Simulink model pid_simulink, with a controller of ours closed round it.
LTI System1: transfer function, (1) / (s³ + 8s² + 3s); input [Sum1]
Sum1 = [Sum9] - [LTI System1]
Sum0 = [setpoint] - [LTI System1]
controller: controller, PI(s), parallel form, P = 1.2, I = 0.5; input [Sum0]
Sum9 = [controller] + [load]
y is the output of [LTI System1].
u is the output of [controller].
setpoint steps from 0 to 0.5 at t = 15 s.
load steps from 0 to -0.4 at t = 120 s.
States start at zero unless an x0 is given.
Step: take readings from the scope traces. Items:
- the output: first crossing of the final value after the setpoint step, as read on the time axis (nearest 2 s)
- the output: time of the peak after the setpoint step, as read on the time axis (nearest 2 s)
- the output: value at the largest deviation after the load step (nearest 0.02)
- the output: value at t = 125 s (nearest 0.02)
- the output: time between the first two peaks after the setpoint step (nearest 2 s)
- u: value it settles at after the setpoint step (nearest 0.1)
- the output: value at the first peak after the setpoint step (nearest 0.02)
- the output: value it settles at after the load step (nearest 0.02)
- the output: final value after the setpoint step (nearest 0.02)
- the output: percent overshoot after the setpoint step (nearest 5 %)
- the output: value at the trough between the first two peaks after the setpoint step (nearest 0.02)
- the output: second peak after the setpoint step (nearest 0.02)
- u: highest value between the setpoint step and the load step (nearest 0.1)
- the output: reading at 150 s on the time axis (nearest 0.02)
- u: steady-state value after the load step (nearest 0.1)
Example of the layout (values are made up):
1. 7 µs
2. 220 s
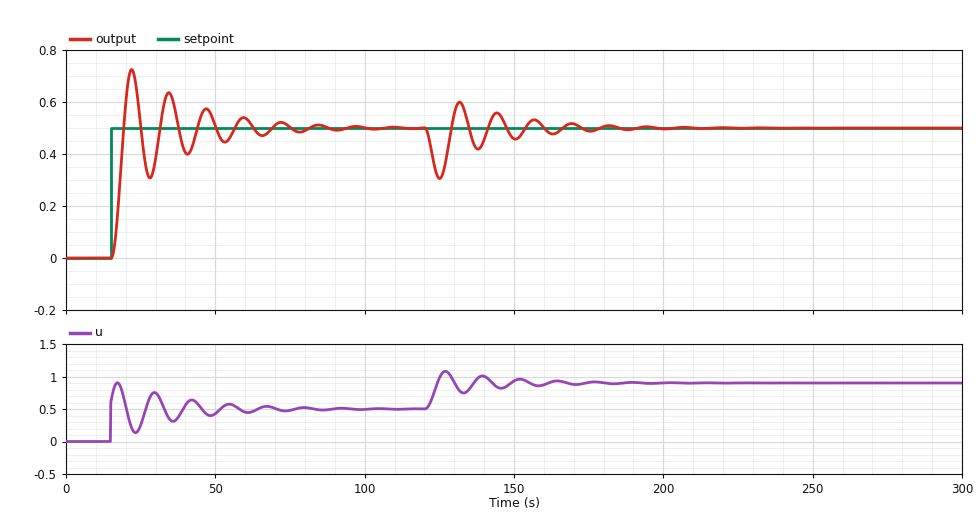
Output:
1. 20 s
2. 22 s
3. 0.30
4. 0.30
5. 12 s
6. 0.5
7. 0.72
8. 0.50
9. 0.50
10. 45 %
11. 0.30
12. 0.64
13. 0.9
14. 0.46
15. 0.9
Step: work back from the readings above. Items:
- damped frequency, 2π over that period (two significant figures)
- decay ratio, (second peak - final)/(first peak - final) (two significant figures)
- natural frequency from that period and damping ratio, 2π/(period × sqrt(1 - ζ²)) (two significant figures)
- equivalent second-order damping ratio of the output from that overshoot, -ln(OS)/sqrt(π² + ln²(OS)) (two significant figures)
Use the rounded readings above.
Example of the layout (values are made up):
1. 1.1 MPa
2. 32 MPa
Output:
1. 0.52 rad/s
2. 0.64
3. 0.54 rad/s
4. 0.25
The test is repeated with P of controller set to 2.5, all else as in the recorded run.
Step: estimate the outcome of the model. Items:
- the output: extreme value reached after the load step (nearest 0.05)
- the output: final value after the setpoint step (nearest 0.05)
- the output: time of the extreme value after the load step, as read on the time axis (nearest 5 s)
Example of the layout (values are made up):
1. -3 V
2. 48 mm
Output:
1. 0.35
2. 0.50
3. 125 s
